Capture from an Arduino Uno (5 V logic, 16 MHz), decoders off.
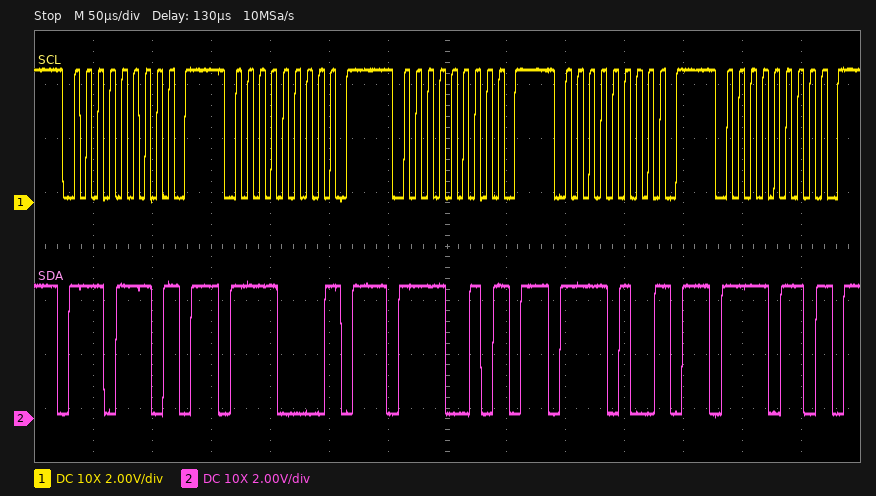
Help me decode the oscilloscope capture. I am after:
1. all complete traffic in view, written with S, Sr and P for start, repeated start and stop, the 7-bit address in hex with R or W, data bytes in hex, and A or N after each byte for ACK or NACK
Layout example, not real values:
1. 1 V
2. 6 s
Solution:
1. S 77W N P S 78W N P S 79W N P S 7AW N P S 7BW N P
